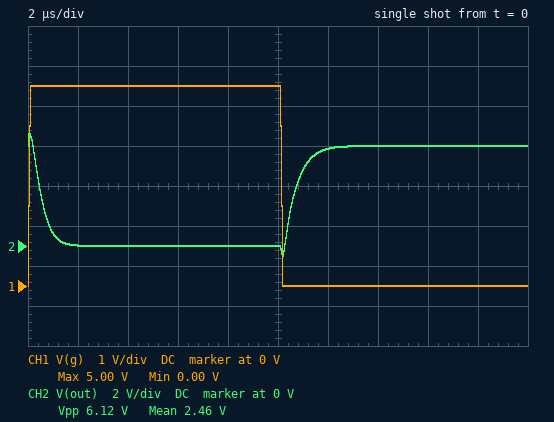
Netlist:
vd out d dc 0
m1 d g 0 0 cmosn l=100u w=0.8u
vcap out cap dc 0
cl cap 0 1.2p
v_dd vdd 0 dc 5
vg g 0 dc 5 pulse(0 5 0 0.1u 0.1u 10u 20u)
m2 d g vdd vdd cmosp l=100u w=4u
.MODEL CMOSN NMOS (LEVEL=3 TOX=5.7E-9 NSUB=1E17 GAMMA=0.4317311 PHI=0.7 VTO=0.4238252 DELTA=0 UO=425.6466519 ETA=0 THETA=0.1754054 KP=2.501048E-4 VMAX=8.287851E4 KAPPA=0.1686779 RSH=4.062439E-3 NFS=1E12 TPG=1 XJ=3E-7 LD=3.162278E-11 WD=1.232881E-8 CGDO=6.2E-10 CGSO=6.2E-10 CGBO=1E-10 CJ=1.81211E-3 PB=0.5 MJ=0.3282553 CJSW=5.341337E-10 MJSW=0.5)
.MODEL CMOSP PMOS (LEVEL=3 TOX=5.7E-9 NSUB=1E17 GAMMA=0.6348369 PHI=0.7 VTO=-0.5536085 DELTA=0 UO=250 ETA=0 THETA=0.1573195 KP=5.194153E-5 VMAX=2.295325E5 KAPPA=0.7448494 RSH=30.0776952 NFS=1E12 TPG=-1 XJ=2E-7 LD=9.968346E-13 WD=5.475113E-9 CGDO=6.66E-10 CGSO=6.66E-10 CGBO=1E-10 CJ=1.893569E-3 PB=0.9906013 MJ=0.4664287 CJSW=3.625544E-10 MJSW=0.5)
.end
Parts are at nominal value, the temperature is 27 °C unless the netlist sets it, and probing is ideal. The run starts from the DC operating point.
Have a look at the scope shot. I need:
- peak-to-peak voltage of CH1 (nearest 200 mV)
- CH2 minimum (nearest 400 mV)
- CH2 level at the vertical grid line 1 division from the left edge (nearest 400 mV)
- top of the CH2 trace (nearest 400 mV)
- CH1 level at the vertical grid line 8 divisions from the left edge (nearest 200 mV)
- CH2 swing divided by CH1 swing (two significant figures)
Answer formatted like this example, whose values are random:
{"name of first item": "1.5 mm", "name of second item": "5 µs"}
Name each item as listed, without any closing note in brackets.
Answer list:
{"peak-to-peak voltage of CH1": "5.0 V", "CH2 minimum": "-400 mV", "CH2 level at the vertical grid line 1 division from the left edge": "0 V", "top of the CH2 trace": "5.6 V", "CH1 level at the vertical grid line 8 divisions from the left edge": "0 V", "CH2 swing divided by CH1 swing": "1.2"}
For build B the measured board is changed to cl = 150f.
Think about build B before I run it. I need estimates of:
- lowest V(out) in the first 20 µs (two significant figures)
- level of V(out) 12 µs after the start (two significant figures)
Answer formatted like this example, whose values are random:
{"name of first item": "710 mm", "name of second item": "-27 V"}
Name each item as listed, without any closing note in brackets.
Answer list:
{"lowest V(out) in the first 20 µs": "-540 mV", "level of V(out) 12 µs after the start": "5.0 V"}
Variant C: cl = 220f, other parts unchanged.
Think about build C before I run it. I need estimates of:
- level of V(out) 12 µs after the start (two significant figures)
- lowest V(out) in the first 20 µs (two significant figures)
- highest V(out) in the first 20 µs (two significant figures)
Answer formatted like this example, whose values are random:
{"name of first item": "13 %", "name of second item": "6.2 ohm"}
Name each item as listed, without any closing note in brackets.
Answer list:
{"level of V(out) 12 µs after the start": "5.0 V", "lowest V(out) in the first 20 µs": "-540 mV", "highest V(out) in the first 20 µs": "5.6 V"}
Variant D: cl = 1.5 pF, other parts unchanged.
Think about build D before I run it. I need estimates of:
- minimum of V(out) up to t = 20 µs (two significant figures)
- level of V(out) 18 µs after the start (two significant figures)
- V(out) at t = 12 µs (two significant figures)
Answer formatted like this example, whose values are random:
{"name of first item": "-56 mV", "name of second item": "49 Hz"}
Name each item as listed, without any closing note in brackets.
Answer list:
{"minimum of V(out) up to t = 20 µs": "-500 mV", "level of V(out) 18 µs after the start": "5.0 V", "V(out) at t = 12 µs": "4.8 V"}
